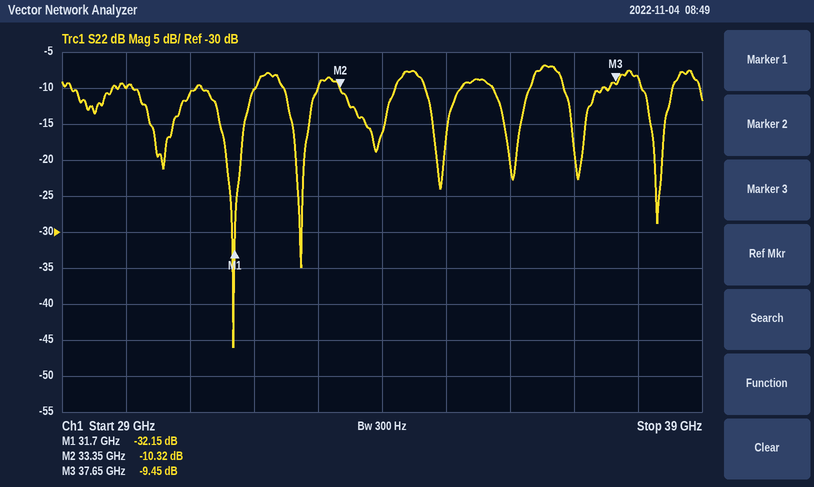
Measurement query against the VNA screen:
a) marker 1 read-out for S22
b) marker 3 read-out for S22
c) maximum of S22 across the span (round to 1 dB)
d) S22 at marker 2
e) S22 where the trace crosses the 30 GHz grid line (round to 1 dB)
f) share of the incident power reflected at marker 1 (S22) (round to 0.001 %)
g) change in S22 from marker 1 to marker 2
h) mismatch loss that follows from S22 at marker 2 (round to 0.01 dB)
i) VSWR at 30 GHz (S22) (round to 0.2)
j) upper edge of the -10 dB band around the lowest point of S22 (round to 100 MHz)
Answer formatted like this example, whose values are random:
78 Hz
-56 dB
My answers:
-32.15 dB
-9.45 dB
-7 dB
-10.32 dB
-10 dB
0.061 %
21.83 dB
0.42 dB
2.0
32.0 GHz
